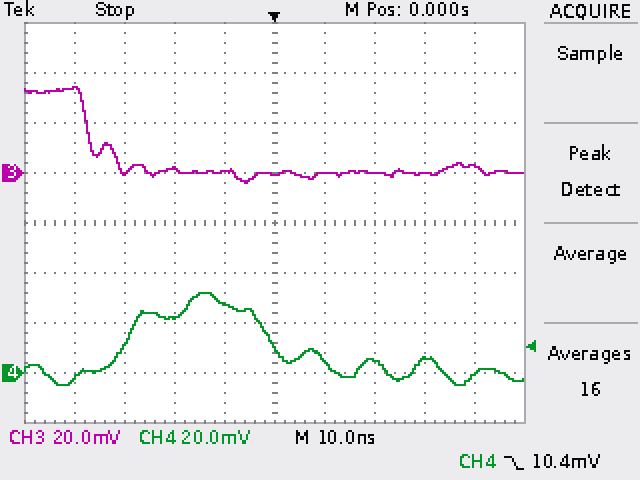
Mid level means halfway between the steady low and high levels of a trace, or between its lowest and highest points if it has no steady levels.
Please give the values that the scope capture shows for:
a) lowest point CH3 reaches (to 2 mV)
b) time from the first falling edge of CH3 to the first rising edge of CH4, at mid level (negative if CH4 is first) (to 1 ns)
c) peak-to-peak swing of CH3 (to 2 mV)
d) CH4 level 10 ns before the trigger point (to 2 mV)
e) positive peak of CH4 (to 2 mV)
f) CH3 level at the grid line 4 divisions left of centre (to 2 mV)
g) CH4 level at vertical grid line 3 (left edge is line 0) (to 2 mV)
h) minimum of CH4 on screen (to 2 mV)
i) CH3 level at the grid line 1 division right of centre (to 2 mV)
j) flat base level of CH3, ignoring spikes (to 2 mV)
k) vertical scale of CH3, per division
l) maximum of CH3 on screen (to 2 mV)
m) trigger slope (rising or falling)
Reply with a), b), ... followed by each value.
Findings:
a) -4 mV
b) +8 ns
c) 38 mV
d) 28 mV
e) 32 mV
f) 34 mV
g) 22 mV
h) -4 mV
i) 0 mV
j) 0 mV
k) 20 mV
l) 34 mV
m) falling
